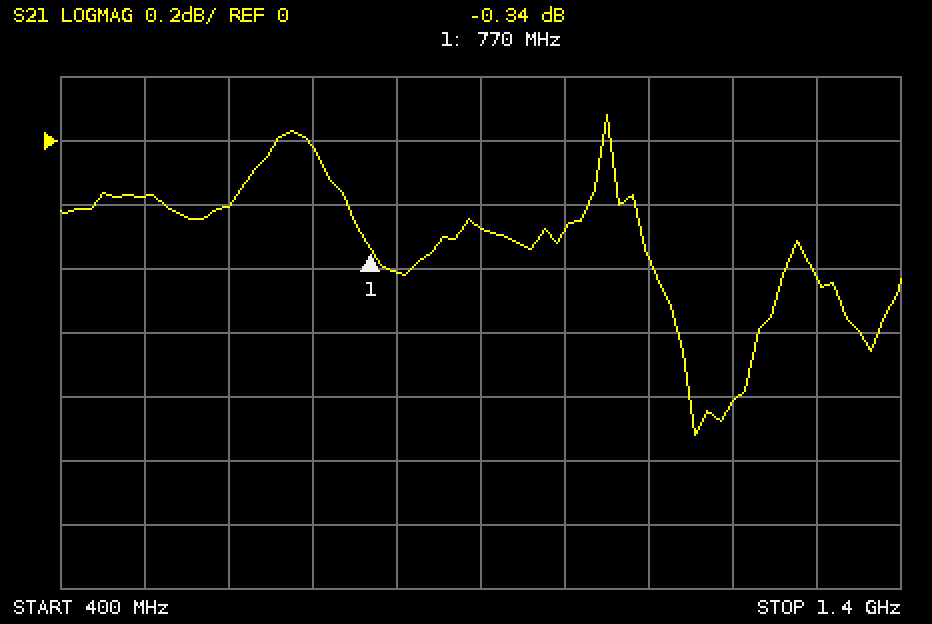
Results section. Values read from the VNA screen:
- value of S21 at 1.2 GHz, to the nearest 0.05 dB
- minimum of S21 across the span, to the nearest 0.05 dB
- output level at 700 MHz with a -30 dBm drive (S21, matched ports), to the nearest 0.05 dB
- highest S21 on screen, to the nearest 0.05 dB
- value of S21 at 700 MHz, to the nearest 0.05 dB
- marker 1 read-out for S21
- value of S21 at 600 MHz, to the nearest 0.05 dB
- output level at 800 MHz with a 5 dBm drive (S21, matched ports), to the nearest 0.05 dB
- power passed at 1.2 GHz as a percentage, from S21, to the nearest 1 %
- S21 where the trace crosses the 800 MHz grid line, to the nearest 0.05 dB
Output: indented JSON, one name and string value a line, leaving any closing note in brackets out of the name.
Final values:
{
  "value of S21 at 1.2 GHz, to the nearest 0.05 dB": "-0.80 dB",
  "minimum of S21 across the span, to the nearest 0.05 dB": "-0.90 dB",
  "output level at 700 MHz with a -30 dBm drive (S21, matched ports), to the nearest 0.05 dB": "-30.00 dBm",
  "highest S21 on screen, to the nearest 0.05 dB": "0.10 dB",
  "value of S21 at 700 MHz, to the nearest 0.05 dB": "0.00 dB",
  "marker 1 read-out for S21": "-0.34 dB",
  "value of S21 at 600 MHz, to the nearest 0.05 dB": "-0.20 dB",
  "output level at 800 MHz with a 5 dBm drive (S21, matched ports), to the nearest 0.05 dB": "4.60 dBm",
  "power passed at 1.2 GHz as a percentage, from S21, to the nearest 1 %": "83 %",
  "S21 where the trace crosses the 800 MHz grid line, to the nearest 0.05 dB": "-0.40 dB"
}
